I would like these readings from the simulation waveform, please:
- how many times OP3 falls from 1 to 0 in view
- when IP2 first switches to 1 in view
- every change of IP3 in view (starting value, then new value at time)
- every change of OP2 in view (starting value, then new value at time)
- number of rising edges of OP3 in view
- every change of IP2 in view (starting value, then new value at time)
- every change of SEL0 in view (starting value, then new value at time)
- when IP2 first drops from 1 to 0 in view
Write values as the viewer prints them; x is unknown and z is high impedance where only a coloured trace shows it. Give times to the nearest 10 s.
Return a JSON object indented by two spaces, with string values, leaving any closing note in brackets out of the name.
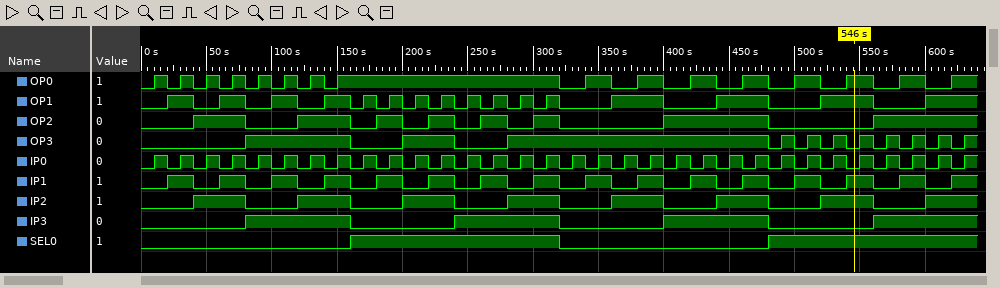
{
  "how many times OP3 falls from 1 to 0 in view": "10",
  "when IP2 first switches to 1 in view": "40 s",
  "every change of IP3 in view": "0, 1 at 80 s, 0 at 160 s, 1 at 240 s, 0 at 320 s, 1 at 400 s, 0 at 480 s, 1 at 560 s",
  "every change of OP2 in view": "0, 1 at 40 s, 0 at 80 s, 1 at 120 s, 0 at 160 s, 1 at 180 s, 0 at 200 s, 1 at 220 s, 0 at 240 s, 1 at 260 s, 0 at 280 s, 1 at 300 s, 0 at 320 s, 1 at 400 s, 0 at 480 s, 1 at 560 s",
  "number of rising edges of OP3 in view": "11",
  "every change of IP2 in view": "0, 1 at 40 s, 0 at 80 s, 1 at 120 s, 0 at 160 s, 1 at 200 s, 0 at 240 s, 1 at 280 s, 0 at 320 s, 1 at 360 s, 0 at 400 s, 1 at 440 s, 0 at 480 s, 1 at 520 s, 0 at 560 s, 1 at 600 s",
  "every change of SEL0 in view": "0, 1 at 160 s, 0 at 320 s, 1 at 480 s",
  "when IP2 first drops from 1 to 0 in view": "80 s"
}
